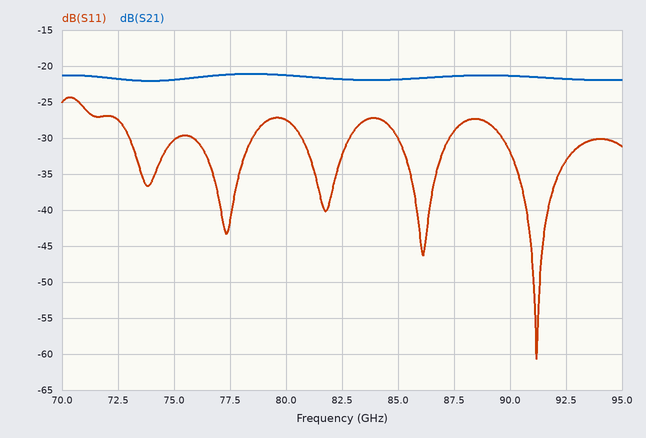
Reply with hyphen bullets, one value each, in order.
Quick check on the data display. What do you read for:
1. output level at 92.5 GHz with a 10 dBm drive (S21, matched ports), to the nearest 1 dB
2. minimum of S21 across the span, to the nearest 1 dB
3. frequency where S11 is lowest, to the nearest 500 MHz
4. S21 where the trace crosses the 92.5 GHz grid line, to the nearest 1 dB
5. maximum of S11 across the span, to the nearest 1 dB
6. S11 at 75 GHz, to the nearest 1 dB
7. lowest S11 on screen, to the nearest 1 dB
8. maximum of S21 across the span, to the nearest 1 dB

- -12 dBm
- -22 dB
- 91.0 GHz
- -22 dB
- -24 dB
- -30 dB
- -61 dB
- -21 dB
